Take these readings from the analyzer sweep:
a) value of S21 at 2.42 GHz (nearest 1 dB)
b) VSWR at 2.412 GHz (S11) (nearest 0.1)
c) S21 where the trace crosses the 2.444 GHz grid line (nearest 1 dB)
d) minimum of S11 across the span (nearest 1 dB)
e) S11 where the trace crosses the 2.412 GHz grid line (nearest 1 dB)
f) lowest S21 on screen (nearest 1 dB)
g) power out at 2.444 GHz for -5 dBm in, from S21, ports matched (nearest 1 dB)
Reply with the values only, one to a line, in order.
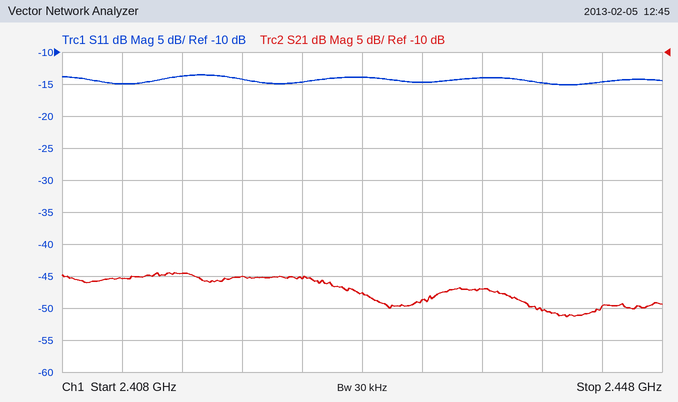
-45 dB
1.4
-50 dB
-15 dB
-15 dB
-51 dB
-55 dBm
